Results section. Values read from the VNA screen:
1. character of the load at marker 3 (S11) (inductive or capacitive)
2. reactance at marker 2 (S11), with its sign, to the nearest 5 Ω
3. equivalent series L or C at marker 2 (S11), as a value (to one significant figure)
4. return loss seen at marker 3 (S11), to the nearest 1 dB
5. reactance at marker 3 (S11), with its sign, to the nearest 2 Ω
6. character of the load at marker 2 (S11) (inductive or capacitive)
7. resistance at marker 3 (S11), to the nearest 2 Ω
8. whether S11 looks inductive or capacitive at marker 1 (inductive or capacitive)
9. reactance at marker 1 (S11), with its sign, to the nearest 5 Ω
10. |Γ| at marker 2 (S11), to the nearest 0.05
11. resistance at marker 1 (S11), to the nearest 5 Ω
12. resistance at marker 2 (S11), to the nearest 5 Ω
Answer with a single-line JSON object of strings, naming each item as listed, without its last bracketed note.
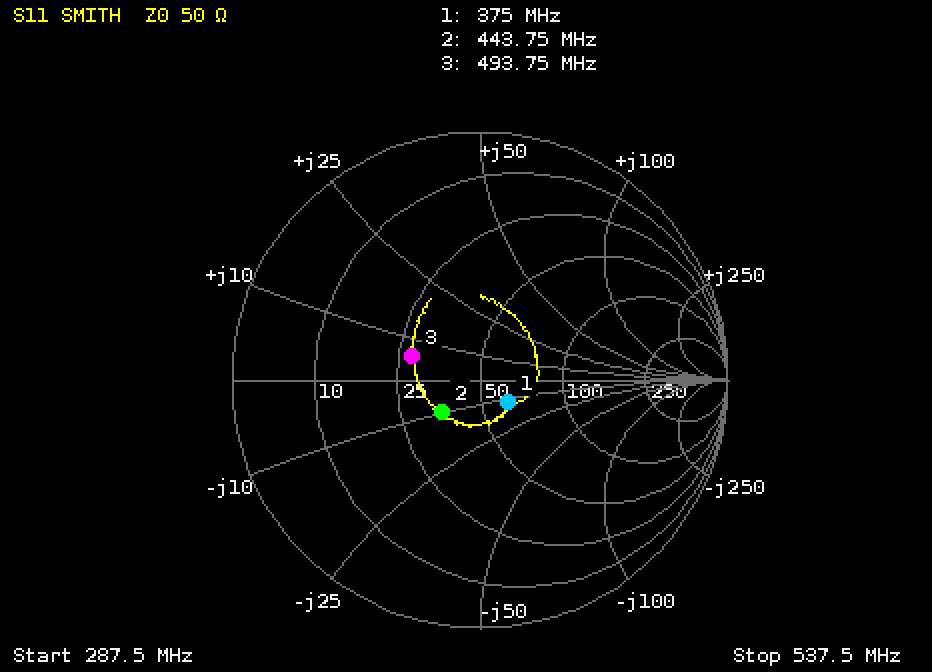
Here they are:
{"character of the load at marker 3 (S11)": "inductive", "reactance at marker 2 (S11), with its sign, to the nearest 5 Ω": "-10 Ω", "equivalent series L or C at marker 2 (S11), as a value": "40 pF", "return loss seen at marker 3 (S11), to the nearest 1 dB": "11 dB", "reactance at marker 3 (S11), with its sign, to the nearest 2 Ω": "+6 Ω", "character of the load at marker 2 (S11)": "capacitive", "resistance at marker 3 (S11), to the nearest 2 Ω": "28 Ω", "whether S11 looks inductive or capacitive at marker 1": "capacitive", "reactance at marker 1 (S11), with its sign, to the nearest 5 Ω": "-10 Ω", "|Γ| at marker 2 (S11), to the nearest 0.05": "0.20", "resistance at marker 1 (S11), to the nearest 5 Ω": "60 Ω", "resistance at marker 2 (S11), to the nearest 5 Ω": "35 Ω"}
